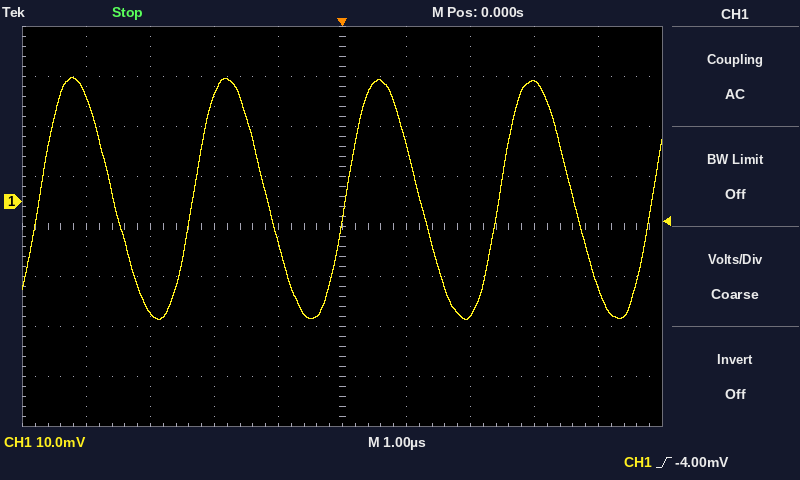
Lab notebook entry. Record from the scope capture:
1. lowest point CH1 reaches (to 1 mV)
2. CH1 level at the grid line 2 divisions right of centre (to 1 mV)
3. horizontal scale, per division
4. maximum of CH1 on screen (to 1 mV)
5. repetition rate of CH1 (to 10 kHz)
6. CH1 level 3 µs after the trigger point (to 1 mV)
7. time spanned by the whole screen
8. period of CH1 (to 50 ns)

-24 mV
-23 mV
1 µs
25 mV
420 kHz
24 mV
10 µs
2.40 µs
